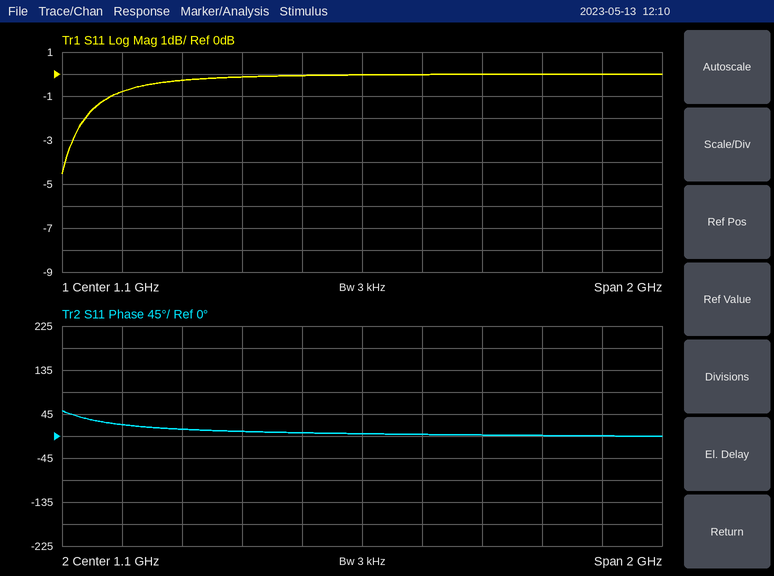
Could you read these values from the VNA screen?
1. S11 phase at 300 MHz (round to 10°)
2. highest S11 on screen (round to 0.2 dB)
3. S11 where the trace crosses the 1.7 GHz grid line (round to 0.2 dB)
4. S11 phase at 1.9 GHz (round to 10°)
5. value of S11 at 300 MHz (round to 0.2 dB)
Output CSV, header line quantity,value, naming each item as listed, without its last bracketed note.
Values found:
quantity,value
S11 phase at 300 MHz,20°
highest S11 on screen,0.0 dB
S11 where the trace crosses the 1.7 GHz grid line,0.0 dB
S11 phase at 1.9 GHz,0°
value of S11 at 300 MHz,-0.8 dB
